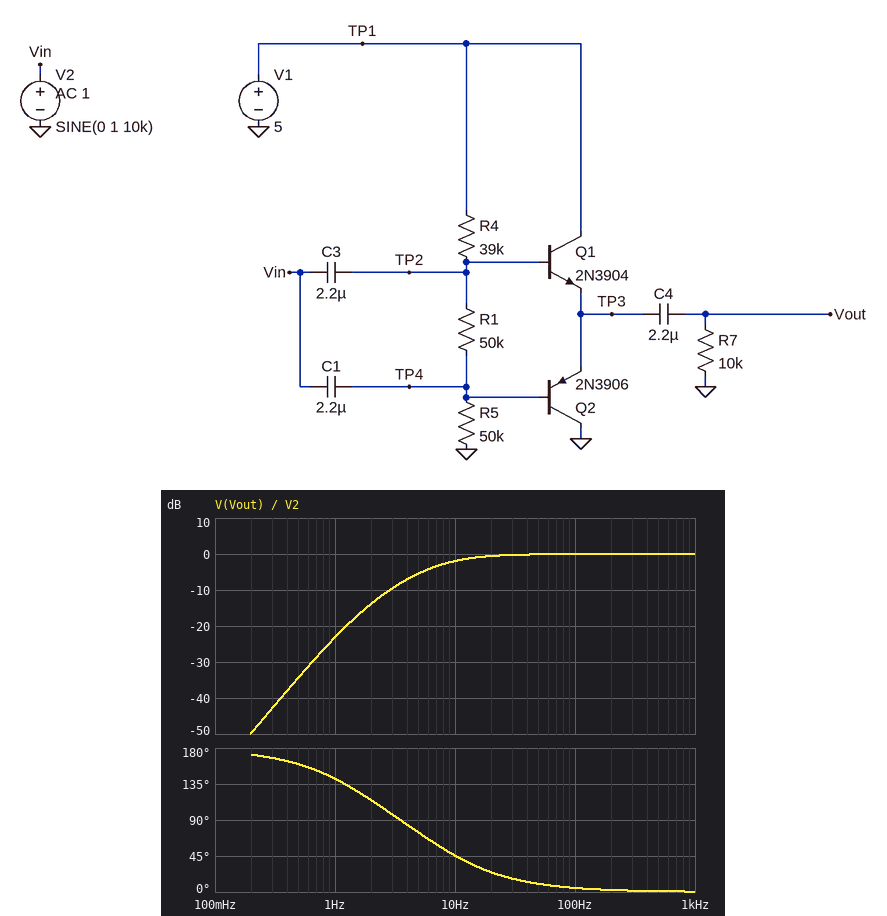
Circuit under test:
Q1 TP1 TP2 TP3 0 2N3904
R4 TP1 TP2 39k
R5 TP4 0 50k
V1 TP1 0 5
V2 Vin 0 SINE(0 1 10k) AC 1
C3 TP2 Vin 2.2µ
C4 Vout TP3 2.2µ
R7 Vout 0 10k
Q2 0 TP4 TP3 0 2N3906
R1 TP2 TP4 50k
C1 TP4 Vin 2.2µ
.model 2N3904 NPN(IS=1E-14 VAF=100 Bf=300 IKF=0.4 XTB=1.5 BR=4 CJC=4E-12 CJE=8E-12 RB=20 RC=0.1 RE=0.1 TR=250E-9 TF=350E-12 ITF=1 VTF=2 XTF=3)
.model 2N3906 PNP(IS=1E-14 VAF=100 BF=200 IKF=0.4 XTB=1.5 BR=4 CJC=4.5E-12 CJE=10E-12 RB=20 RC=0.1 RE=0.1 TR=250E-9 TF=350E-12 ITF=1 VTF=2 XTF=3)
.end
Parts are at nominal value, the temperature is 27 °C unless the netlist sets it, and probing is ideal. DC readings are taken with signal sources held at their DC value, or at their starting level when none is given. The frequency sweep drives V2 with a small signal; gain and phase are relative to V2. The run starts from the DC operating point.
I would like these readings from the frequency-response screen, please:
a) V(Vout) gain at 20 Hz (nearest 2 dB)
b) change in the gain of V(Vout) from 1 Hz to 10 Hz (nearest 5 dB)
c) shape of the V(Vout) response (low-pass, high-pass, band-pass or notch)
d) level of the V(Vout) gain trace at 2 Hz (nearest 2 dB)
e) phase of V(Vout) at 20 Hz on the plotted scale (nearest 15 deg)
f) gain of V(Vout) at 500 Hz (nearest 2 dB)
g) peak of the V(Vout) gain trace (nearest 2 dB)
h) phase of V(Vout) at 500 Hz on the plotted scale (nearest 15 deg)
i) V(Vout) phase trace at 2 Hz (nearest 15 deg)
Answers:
0 dB
20 dB
high-pass
-14 dB
30 deg
0 dB
0 dB
0 deg
120 deg
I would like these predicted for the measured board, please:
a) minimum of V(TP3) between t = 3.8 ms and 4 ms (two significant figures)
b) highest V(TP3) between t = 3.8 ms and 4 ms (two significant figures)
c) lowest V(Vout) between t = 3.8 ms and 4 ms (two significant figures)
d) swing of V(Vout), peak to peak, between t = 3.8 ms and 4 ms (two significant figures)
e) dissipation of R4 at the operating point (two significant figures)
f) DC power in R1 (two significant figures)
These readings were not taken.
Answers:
1.8 V
3.8 V
-1.0 V
2.0 V
56 µW
38 µW
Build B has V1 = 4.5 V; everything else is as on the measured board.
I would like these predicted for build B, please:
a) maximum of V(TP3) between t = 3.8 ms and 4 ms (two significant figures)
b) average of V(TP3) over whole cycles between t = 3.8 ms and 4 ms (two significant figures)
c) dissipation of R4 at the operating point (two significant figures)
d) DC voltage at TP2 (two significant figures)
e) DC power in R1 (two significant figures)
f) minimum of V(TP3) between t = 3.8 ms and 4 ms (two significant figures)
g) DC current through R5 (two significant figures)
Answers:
3.5 V
2.5 V
44 µW
3.2 V
36 µW
1.5 V
37 µA
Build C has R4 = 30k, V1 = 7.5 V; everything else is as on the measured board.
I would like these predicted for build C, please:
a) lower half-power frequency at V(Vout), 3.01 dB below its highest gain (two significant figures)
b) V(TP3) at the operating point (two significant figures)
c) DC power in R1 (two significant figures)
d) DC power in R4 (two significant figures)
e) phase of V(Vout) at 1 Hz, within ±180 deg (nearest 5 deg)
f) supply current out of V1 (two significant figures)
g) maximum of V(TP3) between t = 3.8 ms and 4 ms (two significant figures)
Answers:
7.8 Hz
4.8 V
41 µW
130 µW
145 deg
11 mA
5.8 V
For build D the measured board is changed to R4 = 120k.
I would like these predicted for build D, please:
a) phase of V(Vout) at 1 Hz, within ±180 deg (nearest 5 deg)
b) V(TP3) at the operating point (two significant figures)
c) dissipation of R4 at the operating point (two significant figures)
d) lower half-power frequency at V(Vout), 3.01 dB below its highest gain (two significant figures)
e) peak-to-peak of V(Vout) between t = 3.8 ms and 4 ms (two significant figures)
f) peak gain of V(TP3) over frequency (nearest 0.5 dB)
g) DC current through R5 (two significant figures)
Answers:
125 deg
1.7 V
62 µW
7.2 Hz
1.9 V
-0.5 dB
23 µA
